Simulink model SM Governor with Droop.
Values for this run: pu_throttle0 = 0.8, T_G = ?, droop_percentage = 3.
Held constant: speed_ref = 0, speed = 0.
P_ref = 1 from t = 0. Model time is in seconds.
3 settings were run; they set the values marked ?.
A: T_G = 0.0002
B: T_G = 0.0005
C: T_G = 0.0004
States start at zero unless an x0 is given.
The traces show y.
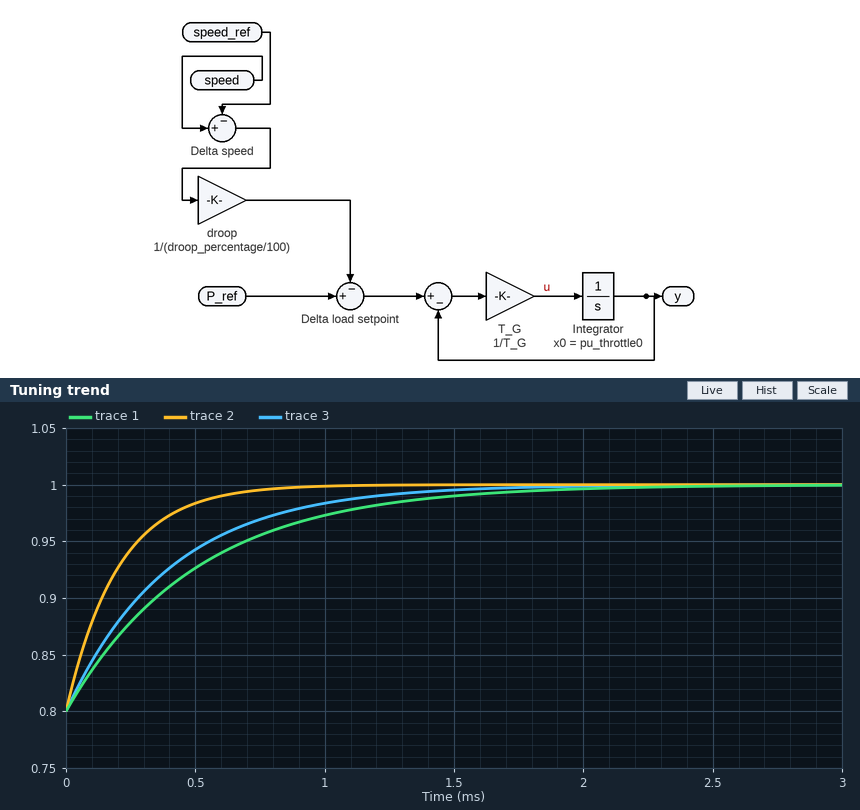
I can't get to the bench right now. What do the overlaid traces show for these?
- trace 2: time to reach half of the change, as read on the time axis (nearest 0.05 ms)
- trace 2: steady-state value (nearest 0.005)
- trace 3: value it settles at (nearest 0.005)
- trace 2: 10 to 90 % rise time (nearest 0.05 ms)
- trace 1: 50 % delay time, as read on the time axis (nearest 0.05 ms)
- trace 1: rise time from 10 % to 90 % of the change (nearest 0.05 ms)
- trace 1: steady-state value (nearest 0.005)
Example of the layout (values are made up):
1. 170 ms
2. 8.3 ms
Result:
1. 0.15 ms
2. 1.000
3. 1.000
4. 0.45 ms
5. 0.35 ms
6. 1.10 ms
7. 1.000
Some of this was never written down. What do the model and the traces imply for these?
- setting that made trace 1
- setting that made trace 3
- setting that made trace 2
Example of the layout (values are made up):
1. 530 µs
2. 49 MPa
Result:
1. B
2. C
3. A
